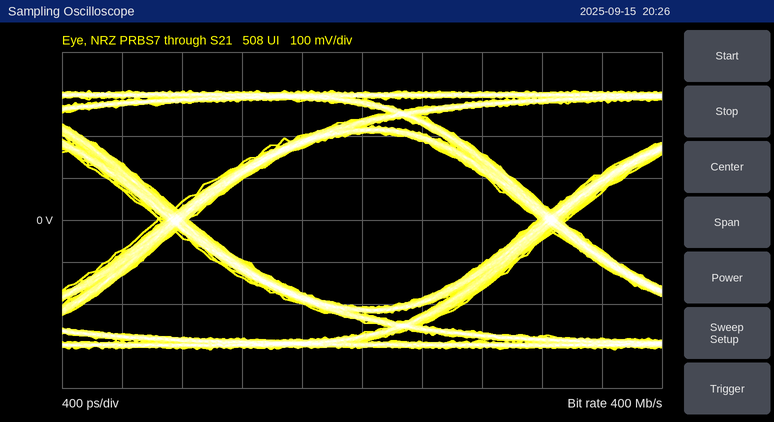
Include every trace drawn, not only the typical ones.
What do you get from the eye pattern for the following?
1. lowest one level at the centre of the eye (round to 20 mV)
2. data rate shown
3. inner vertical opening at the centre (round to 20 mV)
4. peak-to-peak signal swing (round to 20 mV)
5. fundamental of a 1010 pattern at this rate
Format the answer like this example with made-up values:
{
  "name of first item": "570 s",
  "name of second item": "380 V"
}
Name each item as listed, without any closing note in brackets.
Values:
{
  "lowest one level at the centre of the eye": "200 mV",
  "data rate shown": "400 Mb/s",
  "inner vertical opening at the centre": "420 mV",
  "peak-to-peak signal swing": "620 mV",
  "fundamental of a 1010 pattern at this rate": "200 MHz"
}
